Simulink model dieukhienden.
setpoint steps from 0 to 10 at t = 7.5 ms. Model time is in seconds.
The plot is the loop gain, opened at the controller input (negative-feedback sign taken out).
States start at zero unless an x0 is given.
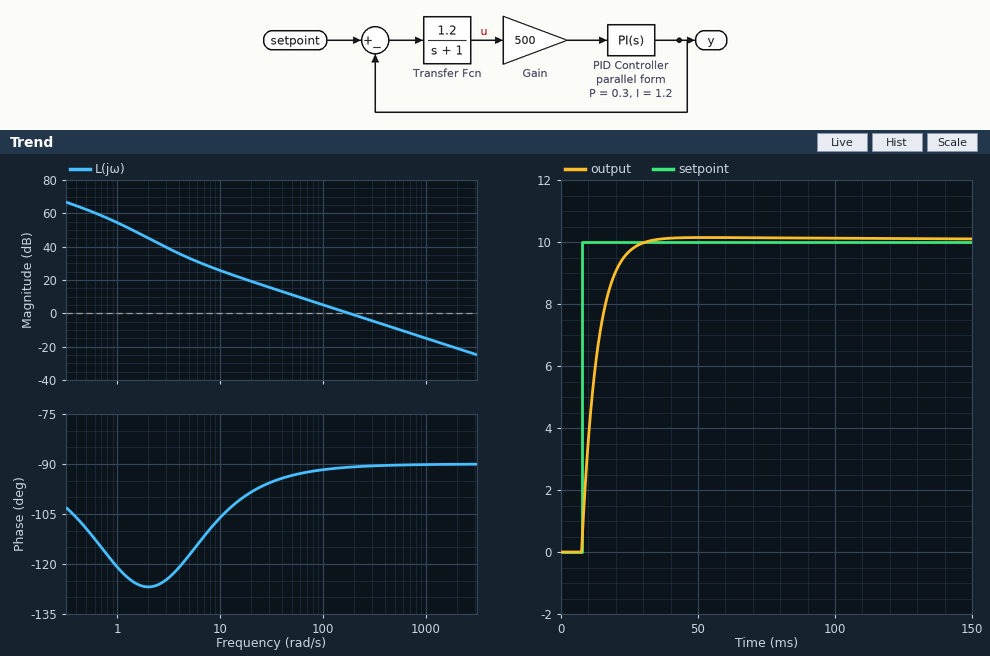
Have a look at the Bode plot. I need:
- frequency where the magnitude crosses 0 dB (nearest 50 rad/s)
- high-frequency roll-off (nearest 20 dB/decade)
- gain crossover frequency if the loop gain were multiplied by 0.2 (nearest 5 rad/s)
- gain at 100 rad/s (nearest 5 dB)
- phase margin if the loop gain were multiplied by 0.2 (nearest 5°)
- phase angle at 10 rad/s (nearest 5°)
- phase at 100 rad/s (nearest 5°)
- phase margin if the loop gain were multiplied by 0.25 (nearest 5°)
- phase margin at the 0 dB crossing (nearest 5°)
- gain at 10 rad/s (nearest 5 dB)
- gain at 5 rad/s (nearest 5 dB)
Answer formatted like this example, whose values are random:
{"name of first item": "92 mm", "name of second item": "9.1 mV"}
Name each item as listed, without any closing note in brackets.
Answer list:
{"frequency where the magnitude crosses 0 dB": "200 rad/s", "high-frequency roll-off": "-20 dB/decade", "gain crossover frequency if the loop gain were multiplied by 0.2": "35 rad/s", "gain at 100 rad/s": "5 dB", "phase margin if the loop gain were multiplied by 0.2": "85°", "phase angle at 10 rad/s": "-105°", "phase at 100 rad/s": "-90°", "phase margin if the loop gain were multiplied by 0.25": "85°", "phase margin at the 0 dB crossing": "90°", "gain at 10 rad/s": "25 dB", "gain at 5 rad/s": "35 dB"}
